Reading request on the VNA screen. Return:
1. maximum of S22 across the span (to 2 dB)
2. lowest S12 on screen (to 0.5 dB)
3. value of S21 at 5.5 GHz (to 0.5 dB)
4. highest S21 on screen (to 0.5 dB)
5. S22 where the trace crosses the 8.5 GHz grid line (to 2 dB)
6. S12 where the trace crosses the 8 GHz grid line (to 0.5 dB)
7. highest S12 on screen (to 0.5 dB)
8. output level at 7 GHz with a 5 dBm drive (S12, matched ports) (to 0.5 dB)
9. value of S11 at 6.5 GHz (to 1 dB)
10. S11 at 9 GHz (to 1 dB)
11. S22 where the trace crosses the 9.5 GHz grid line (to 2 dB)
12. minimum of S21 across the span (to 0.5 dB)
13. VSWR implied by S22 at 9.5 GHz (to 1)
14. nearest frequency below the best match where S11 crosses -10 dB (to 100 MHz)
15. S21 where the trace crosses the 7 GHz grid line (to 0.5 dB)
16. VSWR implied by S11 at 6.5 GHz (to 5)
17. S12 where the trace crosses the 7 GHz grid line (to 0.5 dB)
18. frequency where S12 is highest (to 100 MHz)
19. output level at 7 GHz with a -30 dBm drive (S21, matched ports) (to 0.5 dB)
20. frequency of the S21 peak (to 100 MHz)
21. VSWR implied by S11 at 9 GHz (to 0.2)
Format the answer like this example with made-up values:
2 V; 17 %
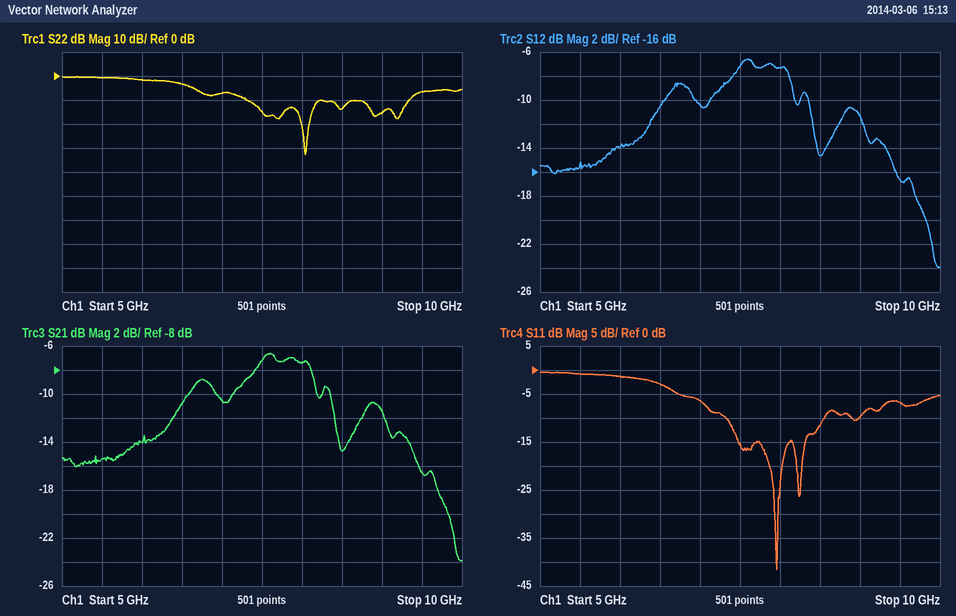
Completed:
0 dB; -24.0 dB; -15.5 dB; -6.5 dB; -14 dB; -7.5 dB; -6.5 dB; -5.5 dBm; -3 dB; -10 dB; -6 dB; -24.0 dB; 3; 7.3 GHz; -10.5 dB; 5; -10.5 dB; 7.6 GHz; -40.5 dBm; 7.6 GHz; 2.0
